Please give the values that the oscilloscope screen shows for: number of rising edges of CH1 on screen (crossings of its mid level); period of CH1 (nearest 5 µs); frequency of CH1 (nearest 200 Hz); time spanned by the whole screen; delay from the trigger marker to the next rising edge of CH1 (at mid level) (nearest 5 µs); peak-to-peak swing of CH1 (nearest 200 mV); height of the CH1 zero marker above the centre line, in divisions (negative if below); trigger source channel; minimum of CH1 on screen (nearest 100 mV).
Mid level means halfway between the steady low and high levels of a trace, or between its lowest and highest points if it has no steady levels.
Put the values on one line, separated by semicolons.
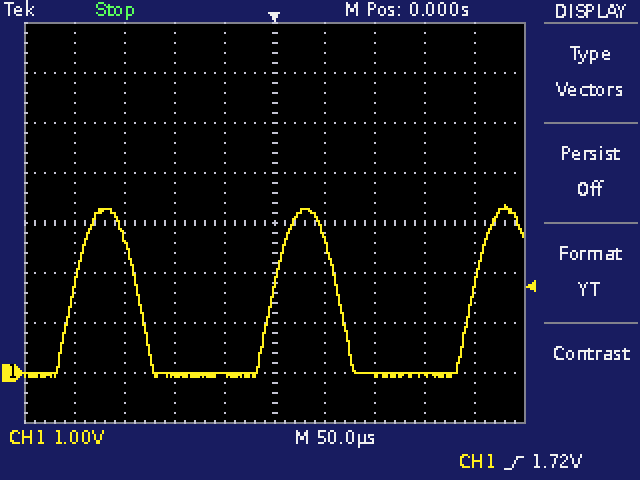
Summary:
3; 200 µs; 5.0 kHz; 500 µs; 200 µs; 3.4 V; -3.0 div; CH1; -100 mV
